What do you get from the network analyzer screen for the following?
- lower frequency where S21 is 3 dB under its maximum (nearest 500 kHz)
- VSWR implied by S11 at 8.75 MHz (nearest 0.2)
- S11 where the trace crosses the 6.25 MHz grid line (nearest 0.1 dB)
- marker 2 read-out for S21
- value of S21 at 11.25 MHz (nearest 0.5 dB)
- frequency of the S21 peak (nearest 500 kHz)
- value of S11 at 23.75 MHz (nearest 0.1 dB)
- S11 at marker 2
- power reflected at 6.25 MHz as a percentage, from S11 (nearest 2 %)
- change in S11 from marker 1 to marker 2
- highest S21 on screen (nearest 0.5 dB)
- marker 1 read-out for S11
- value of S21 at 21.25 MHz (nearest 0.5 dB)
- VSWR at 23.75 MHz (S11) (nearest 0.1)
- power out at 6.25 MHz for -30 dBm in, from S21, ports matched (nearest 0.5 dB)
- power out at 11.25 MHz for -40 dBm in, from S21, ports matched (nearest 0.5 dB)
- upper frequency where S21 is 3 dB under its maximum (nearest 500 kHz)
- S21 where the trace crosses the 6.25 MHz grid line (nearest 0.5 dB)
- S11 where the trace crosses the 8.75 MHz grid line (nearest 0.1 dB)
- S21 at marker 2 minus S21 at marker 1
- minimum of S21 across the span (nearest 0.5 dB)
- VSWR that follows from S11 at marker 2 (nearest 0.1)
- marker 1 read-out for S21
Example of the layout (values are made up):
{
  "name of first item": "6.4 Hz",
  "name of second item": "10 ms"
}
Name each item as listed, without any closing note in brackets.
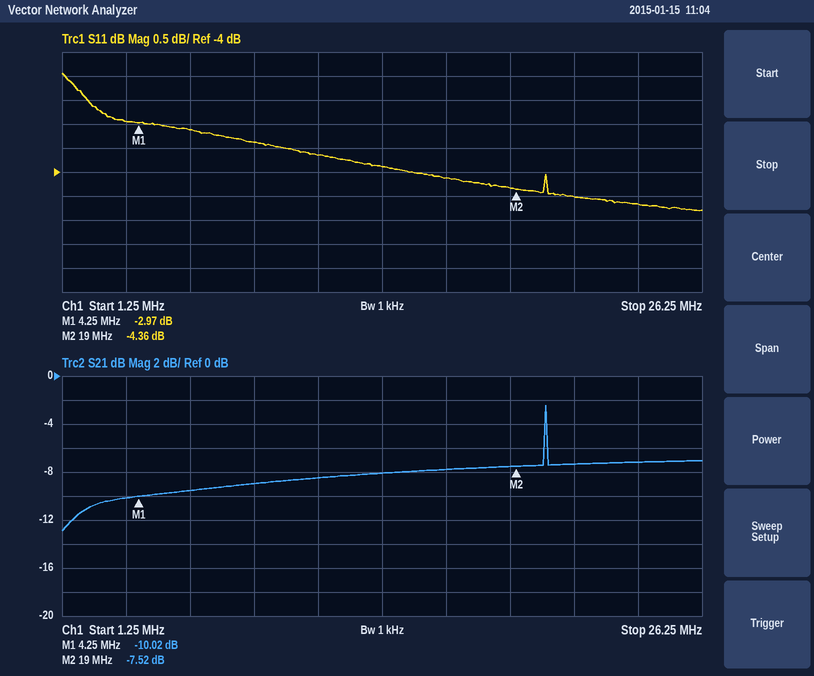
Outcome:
{
  "lower frequency where S21 is 3 dB under its maximum": "20.0 MHz",
  "VSWR implied by S11 at 8.75 MHz": "5.2",
  "S11 where the trace crosses the 6.25 MHz grid line": "-3.1 dB",
  "marker 2 read-out for S21": "-7.52 dB",
  "value of S21 at 11.25 MHz": "-8.5 dB",
  "frequency of the S21 peak": "20.0 MHz",
  "value of S11 at 23.75 MHz": "-4.7 dB",
  "S11 at marker 2": "-4.36 dB",
  "power reflected at 6.25 MHz as a percentage, from S11": "48 %",
  "change in S11 from marker 1 to marker 2": "-1.39 dB",
  "highest S21 on screen": "-2.5 dB",
  "marker 1 read-out for S11": "-2.97 dB",
  "value of S21 at 21.25 MHz": "-7.5 dB",
  "VSWR at 23.75 MHz (S11)": "3.8",
  "power out at 6.25 MHz for -30 dBm in, from S21, ports matched": "-39.5 dBm",
  "power out at 11.25 MHz for -40 dBm in, from S21, ports matched": "-48.5 dBm",
  "upper frequency where S21 is 3 dB under its maximum": "20.0 MHz",
  "S21 where the trace crosses the 6.25 MHz grid line": "-9.5 dB",
  "S11 where the trace crosses the 8.75 MHz grid line": "-3.4 dB",
  "S21 at marker 2 minus S21 at marker 1": "2.50 dB",
  "minimum of S21 across the span": "-13.0 dB",
  "VSWR that follows from S11 at marker 2": "4.1",
  "marker 1 read-out for S21": "-10.02 dB"
}
